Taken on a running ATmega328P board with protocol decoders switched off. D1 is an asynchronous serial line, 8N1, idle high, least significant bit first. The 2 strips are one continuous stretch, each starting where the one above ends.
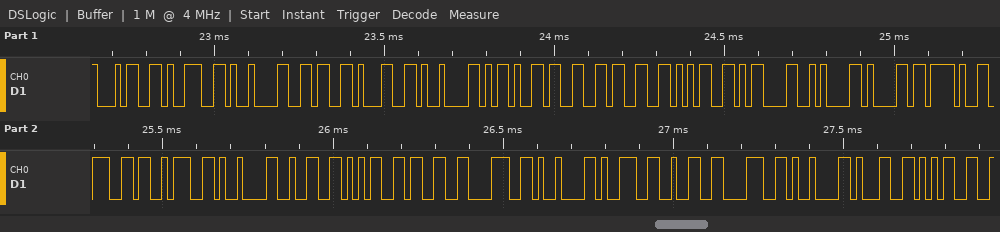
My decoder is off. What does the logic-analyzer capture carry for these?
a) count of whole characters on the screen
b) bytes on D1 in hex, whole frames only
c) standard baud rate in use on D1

28
34 39 09 36 31 09 2D 33 33 35 0D 0A 61 2F 67 3A 09 32 35 33 38 09 39 32 38 09 31 35
57600 baud
